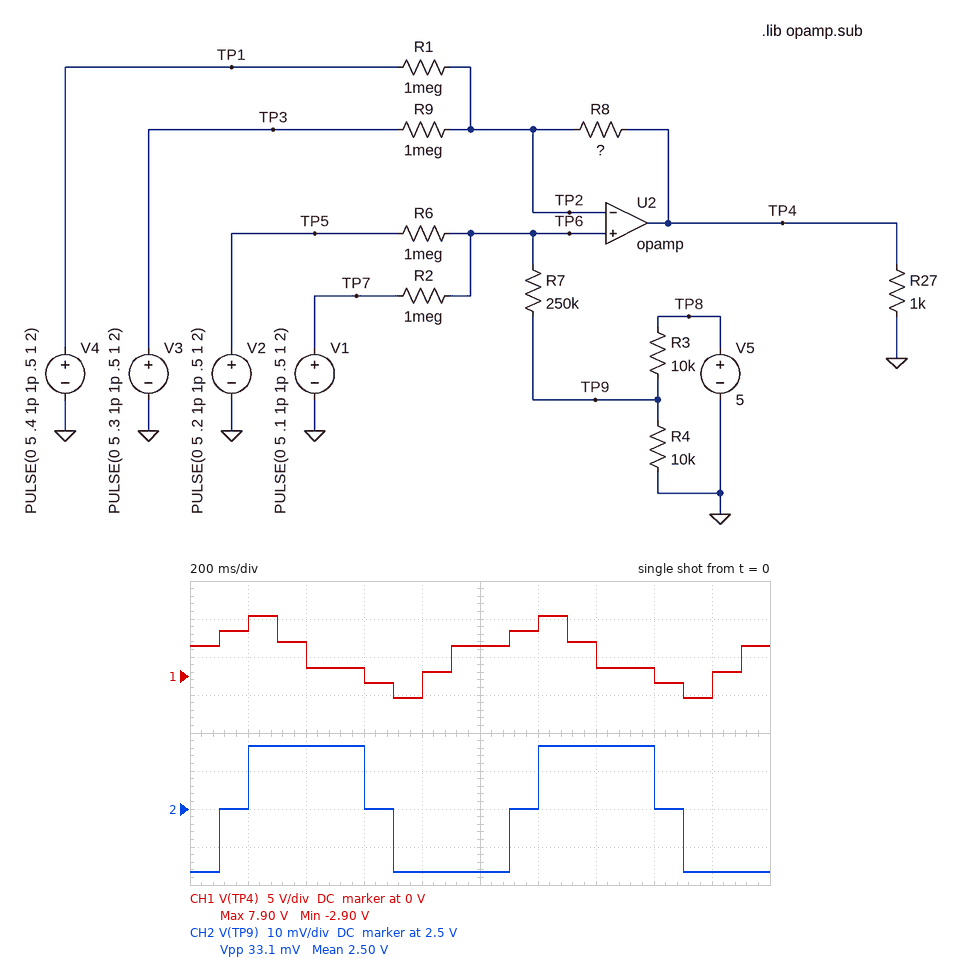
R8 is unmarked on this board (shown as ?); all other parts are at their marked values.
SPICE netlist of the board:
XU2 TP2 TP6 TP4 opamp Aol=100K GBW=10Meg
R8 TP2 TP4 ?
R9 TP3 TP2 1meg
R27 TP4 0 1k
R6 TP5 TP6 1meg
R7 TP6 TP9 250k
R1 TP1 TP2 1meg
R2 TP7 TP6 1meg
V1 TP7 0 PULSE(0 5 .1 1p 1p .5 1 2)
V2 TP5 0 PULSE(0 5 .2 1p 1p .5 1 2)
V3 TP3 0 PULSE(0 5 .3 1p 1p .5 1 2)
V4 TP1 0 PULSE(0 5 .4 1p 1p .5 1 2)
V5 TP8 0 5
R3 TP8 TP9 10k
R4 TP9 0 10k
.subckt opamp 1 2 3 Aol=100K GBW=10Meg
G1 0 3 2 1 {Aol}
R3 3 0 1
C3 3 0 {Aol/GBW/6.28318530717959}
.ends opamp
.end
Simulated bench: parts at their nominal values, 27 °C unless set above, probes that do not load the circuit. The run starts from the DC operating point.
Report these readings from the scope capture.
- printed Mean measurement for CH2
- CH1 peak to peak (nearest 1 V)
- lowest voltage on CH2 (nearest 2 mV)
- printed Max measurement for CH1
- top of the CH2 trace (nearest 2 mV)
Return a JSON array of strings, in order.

["2.50 V", "11 V", "2.484 V", "7.90 V", "2.516 V"]
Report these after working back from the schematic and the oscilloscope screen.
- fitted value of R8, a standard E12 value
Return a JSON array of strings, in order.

["680 kΩ"]
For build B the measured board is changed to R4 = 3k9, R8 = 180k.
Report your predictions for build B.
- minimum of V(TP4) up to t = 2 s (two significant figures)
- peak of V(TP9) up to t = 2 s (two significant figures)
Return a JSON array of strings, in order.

["-530 mV", "1.4 V"]
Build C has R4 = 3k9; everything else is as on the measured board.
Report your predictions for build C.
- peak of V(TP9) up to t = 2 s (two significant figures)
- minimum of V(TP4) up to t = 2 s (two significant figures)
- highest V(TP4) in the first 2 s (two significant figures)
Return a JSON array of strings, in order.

["1.4 V", "-4.6 V", "6.2 V"]
